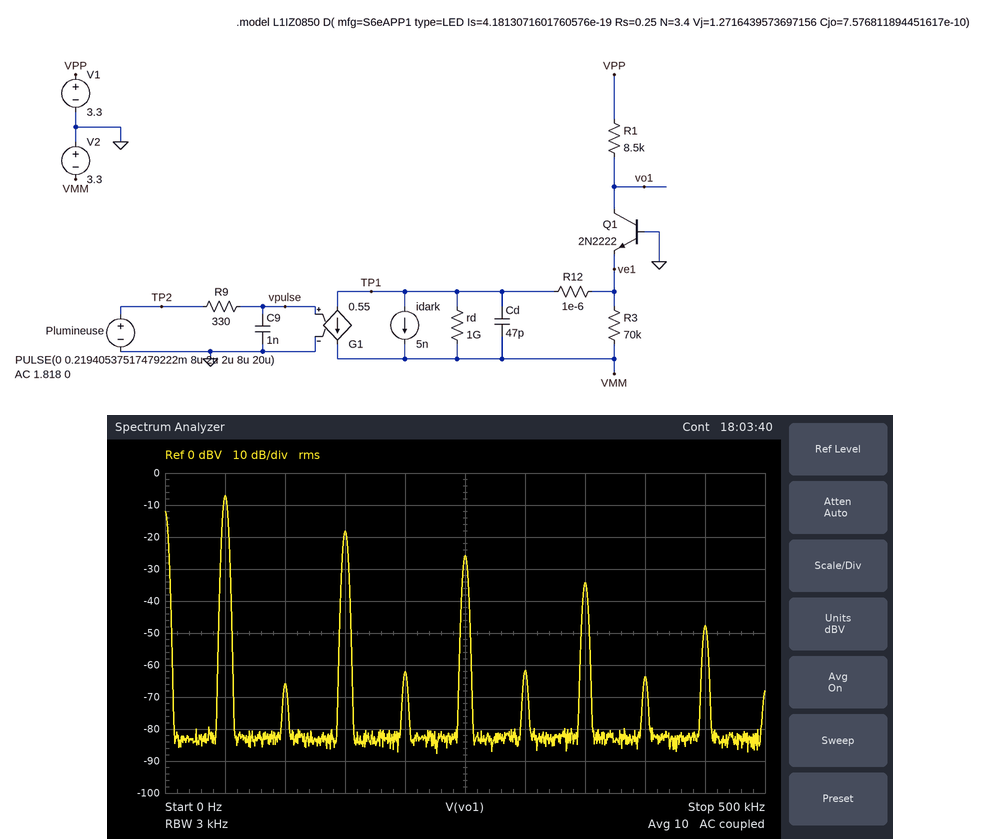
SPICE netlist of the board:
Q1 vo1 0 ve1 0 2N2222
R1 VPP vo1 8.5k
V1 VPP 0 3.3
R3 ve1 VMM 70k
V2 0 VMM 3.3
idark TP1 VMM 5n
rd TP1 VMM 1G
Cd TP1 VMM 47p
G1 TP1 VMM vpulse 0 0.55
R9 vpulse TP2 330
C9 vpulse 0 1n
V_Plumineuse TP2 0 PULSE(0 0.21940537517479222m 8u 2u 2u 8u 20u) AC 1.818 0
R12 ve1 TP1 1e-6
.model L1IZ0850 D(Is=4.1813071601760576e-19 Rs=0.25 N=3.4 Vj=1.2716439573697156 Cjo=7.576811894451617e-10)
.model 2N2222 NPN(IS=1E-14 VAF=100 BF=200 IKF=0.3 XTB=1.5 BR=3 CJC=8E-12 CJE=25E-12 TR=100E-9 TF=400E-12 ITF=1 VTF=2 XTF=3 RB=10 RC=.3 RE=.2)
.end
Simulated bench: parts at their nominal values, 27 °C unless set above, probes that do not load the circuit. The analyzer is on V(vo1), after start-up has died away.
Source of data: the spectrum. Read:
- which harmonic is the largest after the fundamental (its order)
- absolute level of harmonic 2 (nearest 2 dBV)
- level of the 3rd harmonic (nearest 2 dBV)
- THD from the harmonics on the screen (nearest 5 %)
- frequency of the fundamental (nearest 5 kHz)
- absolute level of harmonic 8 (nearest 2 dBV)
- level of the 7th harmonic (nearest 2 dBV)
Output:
3
-66 dBV
-18 dBV
30 %
50 kHz
-64 dBV
-34 dBV
